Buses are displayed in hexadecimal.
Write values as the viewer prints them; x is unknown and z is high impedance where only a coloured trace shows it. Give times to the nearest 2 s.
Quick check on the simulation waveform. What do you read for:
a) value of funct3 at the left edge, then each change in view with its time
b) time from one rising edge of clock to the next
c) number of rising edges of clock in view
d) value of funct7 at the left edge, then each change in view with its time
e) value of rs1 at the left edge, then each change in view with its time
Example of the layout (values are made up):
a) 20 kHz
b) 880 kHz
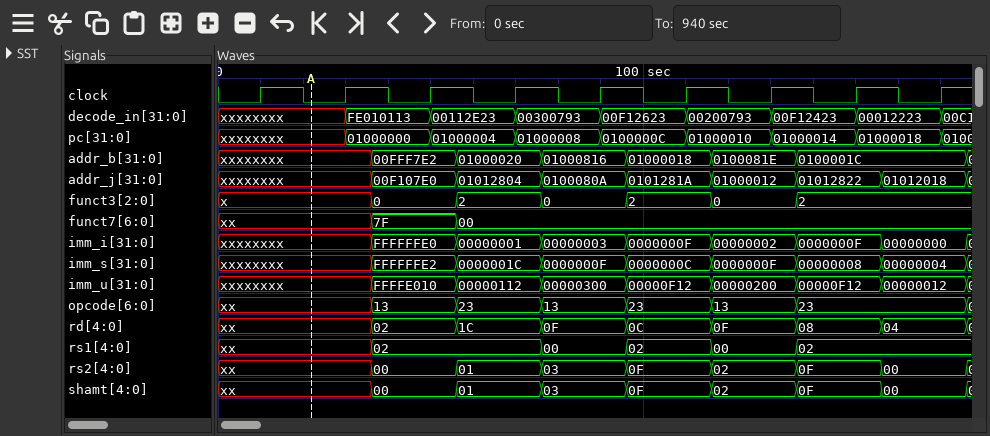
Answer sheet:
a) x, 0 at 36 s, 2 at 56 s, 0 at 76 s, 2 at 96 s, 0 at 116 s, 2 at 136 s
b) 20 s
c) 9
d) xx, 7F at 36 s, 00 at 56 s
e) xx, 02 at 36 s, 00 at 76 s, 02 at 96 s, 00 at 116 s, 02 at 136 s
